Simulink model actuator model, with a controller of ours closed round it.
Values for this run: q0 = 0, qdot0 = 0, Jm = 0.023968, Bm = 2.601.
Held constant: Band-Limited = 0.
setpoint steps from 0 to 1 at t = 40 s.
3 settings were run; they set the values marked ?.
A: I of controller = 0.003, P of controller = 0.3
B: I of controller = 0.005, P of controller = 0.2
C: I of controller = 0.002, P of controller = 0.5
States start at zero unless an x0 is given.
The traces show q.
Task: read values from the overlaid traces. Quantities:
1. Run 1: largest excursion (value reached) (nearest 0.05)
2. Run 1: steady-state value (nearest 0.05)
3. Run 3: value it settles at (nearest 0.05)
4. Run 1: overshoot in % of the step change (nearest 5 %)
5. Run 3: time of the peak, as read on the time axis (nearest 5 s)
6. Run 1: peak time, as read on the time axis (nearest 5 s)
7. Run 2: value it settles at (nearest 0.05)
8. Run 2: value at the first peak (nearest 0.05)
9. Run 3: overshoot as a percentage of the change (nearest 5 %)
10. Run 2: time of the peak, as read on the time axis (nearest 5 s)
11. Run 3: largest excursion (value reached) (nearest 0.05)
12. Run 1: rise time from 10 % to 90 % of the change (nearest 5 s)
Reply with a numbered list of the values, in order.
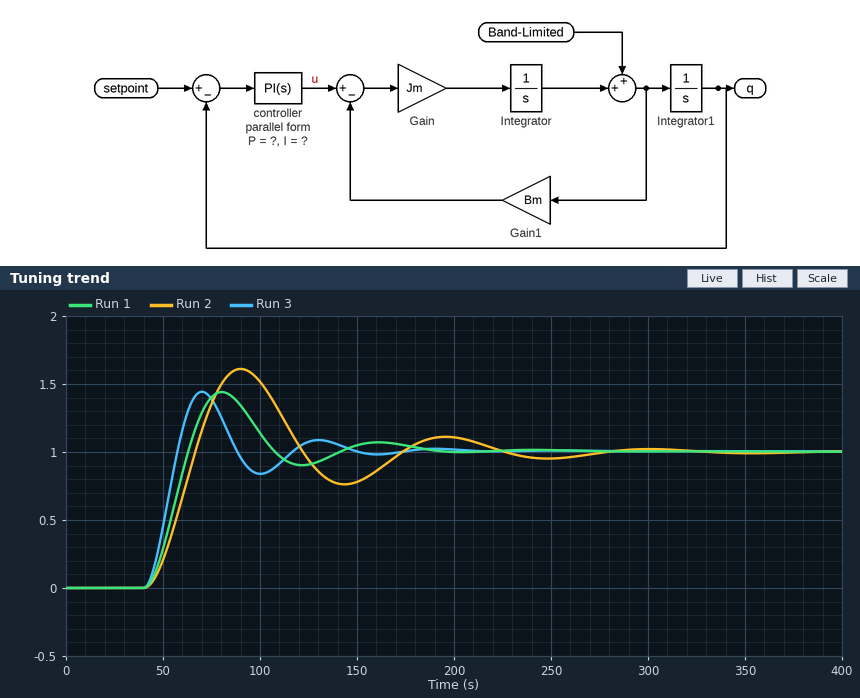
1. 1.45
2. 1.00
3. 1.00
4. 45 %
5. 70 s
6. 80 s
7. 1.00
8. 1.60
9. 45 %
10. 90 s
11. 1.45
12. 15 s
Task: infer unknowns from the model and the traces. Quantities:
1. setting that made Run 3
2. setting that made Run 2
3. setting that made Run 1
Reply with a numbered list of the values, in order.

1. C
2. B
3. A
